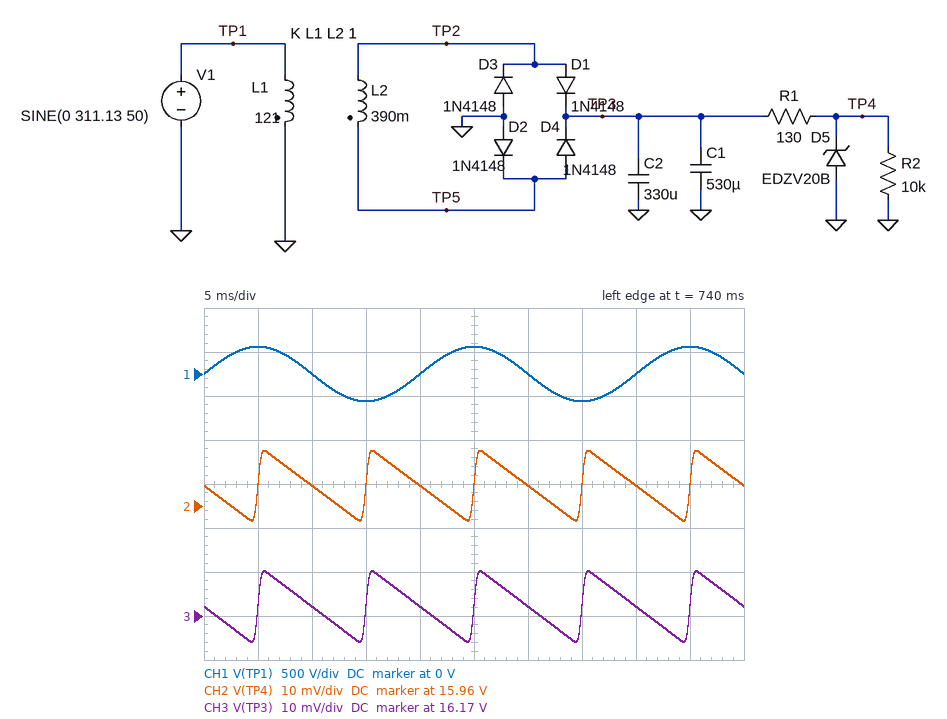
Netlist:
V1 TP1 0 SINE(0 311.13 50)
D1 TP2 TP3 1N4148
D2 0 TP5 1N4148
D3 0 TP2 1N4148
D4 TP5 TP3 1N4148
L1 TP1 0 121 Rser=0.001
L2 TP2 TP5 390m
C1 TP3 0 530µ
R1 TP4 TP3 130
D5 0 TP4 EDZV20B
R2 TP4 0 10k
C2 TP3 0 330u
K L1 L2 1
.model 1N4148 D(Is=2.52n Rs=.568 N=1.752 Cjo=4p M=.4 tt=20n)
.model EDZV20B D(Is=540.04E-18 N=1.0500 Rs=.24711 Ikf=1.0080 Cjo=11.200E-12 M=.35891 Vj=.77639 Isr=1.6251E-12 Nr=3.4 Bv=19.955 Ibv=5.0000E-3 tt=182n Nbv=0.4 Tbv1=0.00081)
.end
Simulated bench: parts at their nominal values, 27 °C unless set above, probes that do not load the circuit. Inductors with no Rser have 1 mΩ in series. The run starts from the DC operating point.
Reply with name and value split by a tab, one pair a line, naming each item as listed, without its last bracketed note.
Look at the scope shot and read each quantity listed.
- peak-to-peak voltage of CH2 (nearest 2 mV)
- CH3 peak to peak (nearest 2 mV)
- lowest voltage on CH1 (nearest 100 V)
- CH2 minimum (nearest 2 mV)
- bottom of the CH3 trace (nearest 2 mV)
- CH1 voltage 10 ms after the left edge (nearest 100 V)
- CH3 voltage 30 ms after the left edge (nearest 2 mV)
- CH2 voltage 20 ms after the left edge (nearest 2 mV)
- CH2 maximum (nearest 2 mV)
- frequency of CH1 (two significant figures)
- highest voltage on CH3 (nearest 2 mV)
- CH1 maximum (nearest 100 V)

peak-to-peak voltage of CH2	16 mV
CH3 peak to peak	16 mV
lowest voltage on CH1	-300 V
CH2 minimum	15.956 V
bottom of the CH3 trace	16.164 V
CH1 voltage 10 ms after the left edge	0 V
CH3 voltage 30 ms after the left edge	16.172 V
CH2 voltage 20 ms after the left edge	15.964 V
CH2 maximum	15.972 V
frequency of CH1	50 Hz
highest voltage on CH3	16.180 V
CH1 maximum	300 V
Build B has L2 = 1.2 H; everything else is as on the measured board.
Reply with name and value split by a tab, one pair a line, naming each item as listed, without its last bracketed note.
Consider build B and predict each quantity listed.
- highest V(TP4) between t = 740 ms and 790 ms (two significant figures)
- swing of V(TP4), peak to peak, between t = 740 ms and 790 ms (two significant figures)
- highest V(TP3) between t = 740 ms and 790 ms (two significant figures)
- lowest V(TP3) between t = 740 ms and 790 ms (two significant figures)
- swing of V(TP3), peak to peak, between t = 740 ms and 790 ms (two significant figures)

highest V(TP4) between t = 740 ms and 790 ms	20 V
swing of V(TP4), peak to peak, between t = 740 ms and 790 ms	2.0 mV
highest V(TP3) between t = 740 ms and 790 ms	29 V
lowest V(TP3) between t = 740 ms and 790 ms	28 V
swing of V(TP3), peak to peak, between t = 740 ms and 790 ms	630 mV
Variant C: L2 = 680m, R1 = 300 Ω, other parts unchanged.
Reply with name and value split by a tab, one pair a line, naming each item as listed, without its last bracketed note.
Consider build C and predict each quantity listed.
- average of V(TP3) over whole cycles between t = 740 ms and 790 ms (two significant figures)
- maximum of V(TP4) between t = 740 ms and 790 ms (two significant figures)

average of V(TP3) over whole cycles between t = 740 ms and 790 ms	22 V
maximum of V(TP4) between t = 740 ms and 790 ms	20 V
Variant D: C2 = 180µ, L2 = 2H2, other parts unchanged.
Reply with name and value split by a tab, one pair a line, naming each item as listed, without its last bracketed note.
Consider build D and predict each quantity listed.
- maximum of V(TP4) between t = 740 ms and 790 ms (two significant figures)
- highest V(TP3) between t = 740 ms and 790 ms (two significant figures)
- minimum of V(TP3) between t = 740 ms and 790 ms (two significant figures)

maximum of V(TP4) between t = 740 ms and 790 ms	20 V
highest V(TP3) between t = 740 ms and 790 ms	39 V
minimum of V(TP3) between t = 740 ms and 790 ms	38 V
